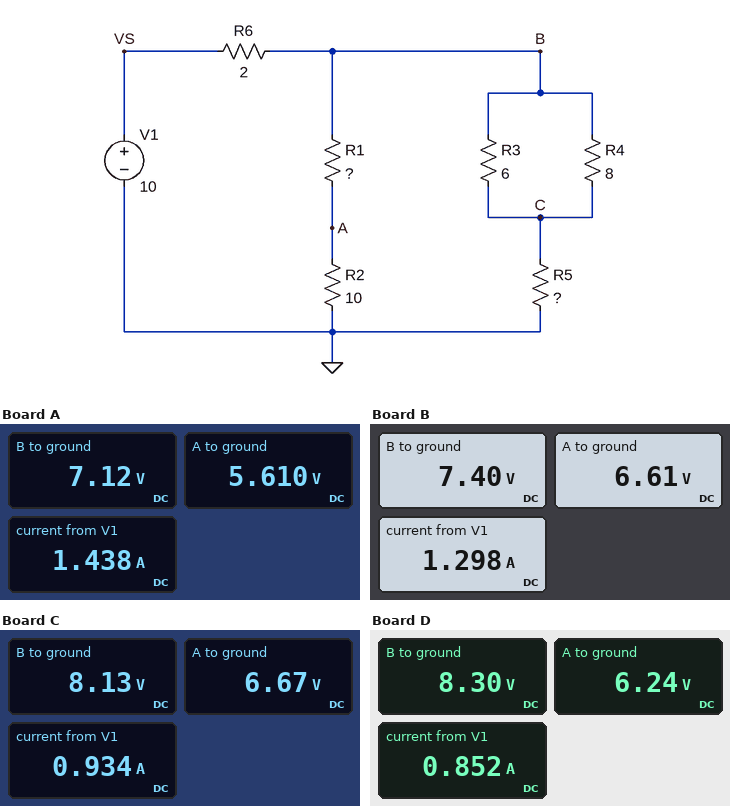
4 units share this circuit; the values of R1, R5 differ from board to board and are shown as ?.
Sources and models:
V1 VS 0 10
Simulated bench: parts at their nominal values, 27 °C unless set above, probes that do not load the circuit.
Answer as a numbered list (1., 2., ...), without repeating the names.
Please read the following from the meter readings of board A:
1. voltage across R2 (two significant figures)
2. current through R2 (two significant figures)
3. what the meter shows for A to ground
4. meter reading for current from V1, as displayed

1. 5.6 V
2. 560 mA
3. 5.610 V
4. 1.438 A
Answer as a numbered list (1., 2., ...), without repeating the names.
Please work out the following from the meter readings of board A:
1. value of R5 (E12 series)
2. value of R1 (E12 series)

1. 4.7 Ω
2. 2.7 Ω
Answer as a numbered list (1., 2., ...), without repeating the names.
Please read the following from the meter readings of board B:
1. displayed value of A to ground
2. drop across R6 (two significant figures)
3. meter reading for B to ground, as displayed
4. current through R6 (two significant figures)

1. 6.61 V
2. 2.6 V
3. 7.40 V
4. 1.3 A
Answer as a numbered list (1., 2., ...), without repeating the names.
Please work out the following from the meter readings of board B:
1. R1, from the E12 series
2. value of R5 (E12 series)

1. 1.2 Ω
2. 8.2 Ω
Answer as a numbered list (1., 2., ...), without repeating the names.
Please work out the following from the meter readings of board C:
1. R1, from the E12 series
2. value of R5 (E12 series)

1. 2.2 Ω
2. 27 Ω
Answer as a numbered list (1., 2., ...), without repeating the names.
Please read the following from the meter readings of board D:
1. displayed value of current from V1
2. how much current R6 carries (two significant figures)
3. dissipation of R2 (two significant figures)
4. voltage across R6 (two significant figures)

1. 0.852 A
2. 850 mA
3. 3.9 W
4. 1.7 V
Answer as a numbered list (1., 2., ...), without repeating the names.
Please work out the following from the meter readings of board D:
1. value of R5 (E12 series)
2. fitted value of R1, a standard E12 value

1. 33 Ω
2. 3.3 Ω
